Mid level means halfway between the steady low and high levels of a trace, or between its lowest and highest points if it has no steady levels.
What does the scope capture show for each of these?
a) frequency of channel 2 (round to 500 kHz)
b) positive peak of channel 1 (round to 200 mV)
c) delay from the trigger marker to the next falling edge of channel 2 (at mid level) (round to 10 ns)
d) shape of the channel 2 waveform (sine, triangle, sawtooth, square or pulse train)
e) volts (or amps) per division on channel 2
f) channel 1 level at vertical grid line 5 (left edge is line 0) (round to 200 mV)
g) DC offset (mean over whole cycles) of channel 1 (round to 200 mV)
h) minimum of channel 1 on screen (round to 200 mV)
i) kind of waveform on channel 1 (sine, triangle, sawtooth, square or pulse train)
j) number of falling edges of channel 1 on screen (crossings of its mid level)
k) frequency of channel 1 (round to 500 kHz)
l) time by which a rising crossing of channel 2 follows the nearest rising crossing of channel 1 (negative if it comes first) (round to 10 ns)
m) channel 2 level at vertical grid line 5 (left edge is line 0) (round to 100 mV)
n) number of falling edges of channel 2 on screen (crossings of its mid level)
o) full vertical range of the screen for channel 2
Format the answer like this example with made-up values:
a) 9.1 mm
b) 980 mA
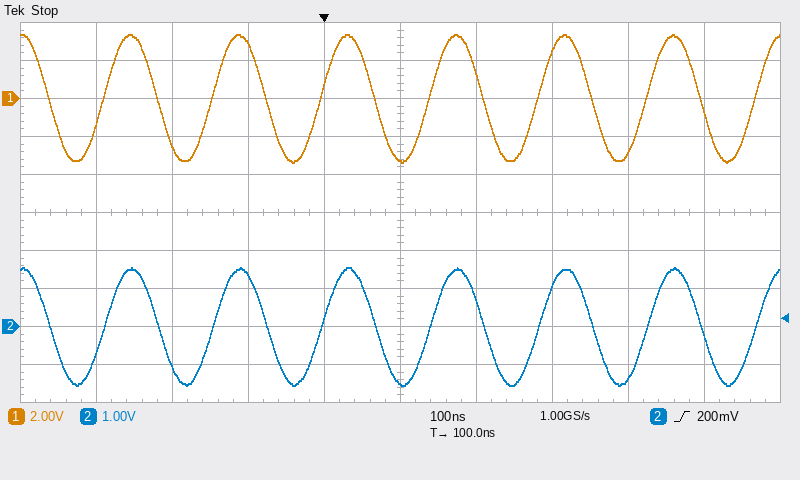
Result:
a) 7.0 MHz
b) 3.4 V
c) 70 ns
d) sine
e) 1 V
f) -3.2 V
g) 0.0 V
h) -3.4 V
i) sine
j) 7
k) 7.0 MHz
l) 0 ns
m) -1.5 V
n) 7
o) 10 V
